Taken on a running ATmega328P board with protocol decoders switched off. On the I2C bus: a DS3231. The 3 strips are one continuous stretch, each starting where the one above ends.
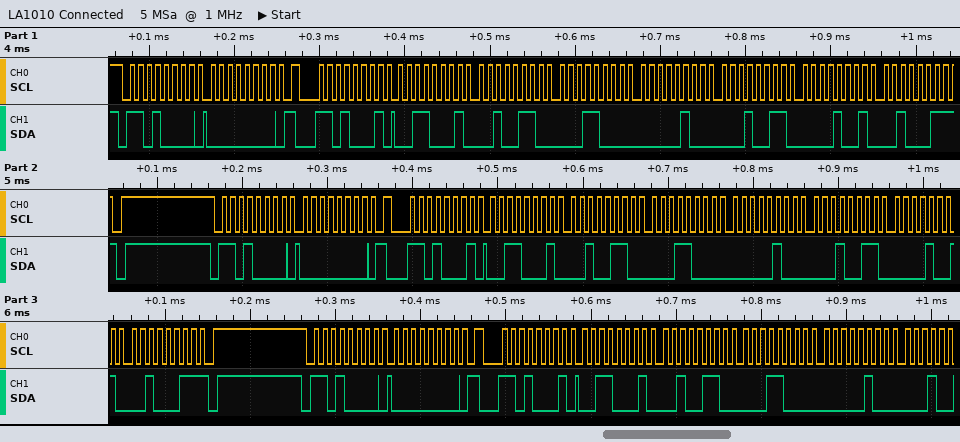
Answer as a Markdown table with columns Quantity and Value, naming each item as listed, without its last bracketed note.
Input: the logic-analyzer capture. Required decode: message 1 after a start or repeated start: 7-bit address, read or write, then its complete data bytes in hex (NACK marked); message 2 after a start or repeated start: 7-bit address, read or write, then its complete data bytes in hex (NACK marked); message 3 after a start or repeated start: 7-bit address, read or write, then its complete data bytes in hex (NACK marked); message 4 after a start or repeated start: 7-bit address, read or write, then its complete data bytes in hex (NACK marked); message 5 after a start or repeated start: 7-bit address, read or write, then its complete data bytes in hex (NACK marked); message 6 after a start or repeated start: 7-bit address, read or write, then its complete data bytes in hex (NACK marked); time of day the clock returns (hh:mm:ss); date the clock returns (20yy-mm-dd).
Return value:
| Quantity | Value |
|---|---|
| message 1 after a start or repeated start: 7-bit address, read or write, then its complete data bytes in hex | 0x68 write: 00 |
| message 2 after a start or repeated start: 7-bit address, read or write, then its complete data bytes in hex | 0x68 read: 31 26 18 04 13 09 23 NACK |
| message 3 after a start or repeated start: 7-bit address, read or write, then its complete data bytes in hex | 0x68 write: 00 |
| message 4 after a start or repeated start: 7-bit address, read or write, then its complete data bytes in hex | 0x68 read: 31 26 18 04 13 09 23 NACK |
| message 5 after a start or repeated start: 7-bit address, read or write, then its complete data bytes in hex | 0x68 write: 00 |
| message 6 after a start or repeated start: 7-bit address, read or write, then its complete data bytes in hex | 0x68 read: 31 26 18 04 |
| time of day the clock returns | 18:26:31 |
| date the clock returns | 2023-09-13 |
